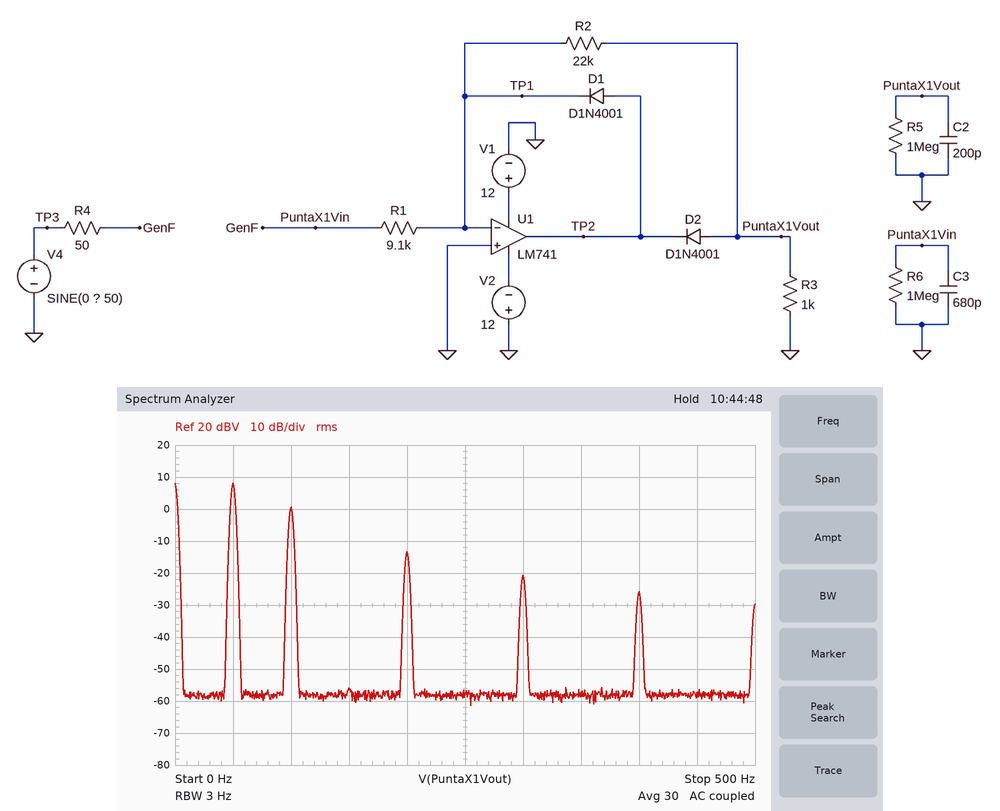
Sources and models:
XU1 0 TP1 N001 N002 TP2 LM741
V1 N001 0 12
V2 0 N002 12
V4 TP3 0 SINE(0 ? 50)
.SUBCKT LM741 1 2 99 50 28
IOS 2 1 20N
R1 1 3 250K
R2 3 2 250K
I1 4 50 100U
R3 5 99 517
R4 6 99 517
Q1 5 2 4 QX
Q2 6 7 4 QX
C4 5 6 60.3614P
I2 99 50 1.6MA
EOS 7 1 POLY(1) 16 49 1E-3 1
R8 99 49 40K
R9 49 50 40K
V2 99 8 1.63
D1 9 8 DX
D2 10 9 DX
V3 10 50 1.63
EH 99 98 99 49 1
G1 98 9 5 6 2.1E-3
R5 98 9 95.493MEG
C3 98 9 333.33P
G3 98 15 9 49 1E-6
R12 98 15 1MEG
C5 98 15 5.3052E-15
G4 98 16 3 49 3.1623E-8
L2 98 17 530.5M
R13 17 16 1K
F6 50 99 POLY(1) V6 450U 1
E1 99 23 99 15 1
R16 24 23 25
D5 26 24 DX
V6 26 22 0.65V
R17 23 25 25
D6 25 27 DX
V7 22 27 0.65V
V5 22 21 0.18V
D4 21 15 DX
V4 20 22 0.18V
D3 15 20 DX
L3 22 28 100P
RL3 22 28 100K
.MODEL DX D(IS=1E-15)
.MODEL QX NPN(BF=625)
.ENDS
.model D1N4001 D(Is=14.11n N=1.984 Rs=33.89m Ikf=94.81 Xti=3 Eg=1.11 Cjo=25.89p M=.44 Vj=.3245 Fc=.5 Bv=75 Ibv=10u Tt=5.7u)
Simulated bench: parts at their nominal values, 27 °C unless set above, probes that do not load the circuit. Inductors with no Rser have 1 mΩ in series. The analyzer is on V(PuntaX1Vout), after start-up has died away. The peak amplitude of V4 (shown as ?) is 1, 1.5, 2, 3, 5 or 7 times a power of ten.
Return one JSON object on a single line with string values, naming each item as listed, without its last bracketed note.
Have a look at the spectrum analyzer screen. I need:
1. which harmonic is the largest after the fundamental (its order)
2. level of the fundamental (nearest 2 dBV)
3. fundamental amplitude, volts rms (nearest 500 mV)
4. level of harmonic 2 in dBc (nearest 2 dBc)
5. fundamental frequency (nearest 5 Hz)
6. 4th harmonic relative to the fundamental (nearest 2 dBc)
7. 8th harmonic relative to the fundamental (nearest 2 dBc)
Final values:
{"which harmonic is the largest after the fundamental": "2", "level of the fundamental": "8 dBV", "fundamental amplitude, volts rms": "2.5 V", "level of harmonic 2 in dBc": "-8 dBc", "fundamental frequency": "50 Hz", "4th harmonic relative to the fundamental": "-22 dBc", "8th harmonic relative to the fundamental": "-34 dBc"}
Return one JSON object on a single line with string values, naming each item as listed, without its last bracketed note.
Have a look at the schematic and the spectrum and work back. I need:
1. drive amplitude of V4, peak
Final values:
{"drive amplitude of V4, peak": "3 V"}
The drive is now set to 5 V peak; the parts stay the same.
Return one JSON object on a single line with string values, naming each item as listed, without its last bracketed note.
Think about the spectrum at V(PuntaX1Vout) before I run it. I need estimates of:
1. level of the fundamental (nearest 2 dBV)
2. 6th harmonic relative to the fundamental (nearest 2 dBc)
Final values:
{"level of the fundamental": "12 dBV", "6th harmonic relative to the fundamental": "-34 dBc"}
